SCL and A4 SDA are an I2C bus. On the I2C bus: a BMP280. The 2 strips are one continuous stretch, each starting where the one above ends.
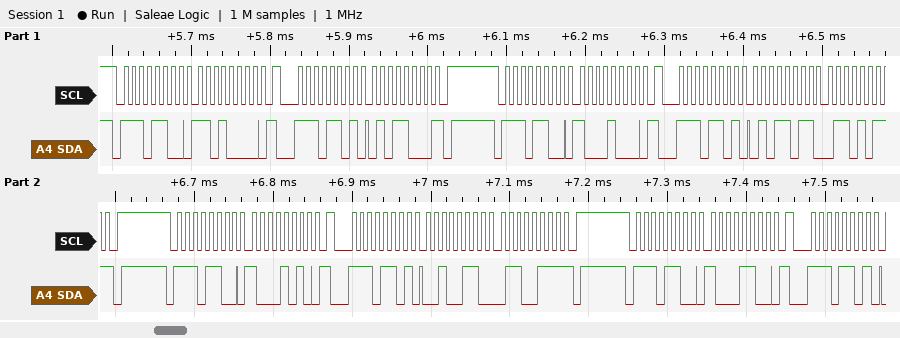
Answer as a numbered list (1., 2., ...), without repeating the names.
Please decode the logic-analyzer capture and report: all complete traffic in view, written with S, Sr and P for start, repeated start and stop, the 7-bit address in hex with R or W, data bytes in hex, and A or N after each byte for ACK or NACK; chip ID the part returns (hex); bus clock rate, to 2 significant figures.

1. S 76W A D0 A Sr 76R A 58 N P S 76W A 88 A Sr 76R A 5B A 6B N P S 76W A 8A A Sr 76R A 26 A 67 N P S 76W A 8C A Sr 76R A
2. 0x58
3. 100 kHz
